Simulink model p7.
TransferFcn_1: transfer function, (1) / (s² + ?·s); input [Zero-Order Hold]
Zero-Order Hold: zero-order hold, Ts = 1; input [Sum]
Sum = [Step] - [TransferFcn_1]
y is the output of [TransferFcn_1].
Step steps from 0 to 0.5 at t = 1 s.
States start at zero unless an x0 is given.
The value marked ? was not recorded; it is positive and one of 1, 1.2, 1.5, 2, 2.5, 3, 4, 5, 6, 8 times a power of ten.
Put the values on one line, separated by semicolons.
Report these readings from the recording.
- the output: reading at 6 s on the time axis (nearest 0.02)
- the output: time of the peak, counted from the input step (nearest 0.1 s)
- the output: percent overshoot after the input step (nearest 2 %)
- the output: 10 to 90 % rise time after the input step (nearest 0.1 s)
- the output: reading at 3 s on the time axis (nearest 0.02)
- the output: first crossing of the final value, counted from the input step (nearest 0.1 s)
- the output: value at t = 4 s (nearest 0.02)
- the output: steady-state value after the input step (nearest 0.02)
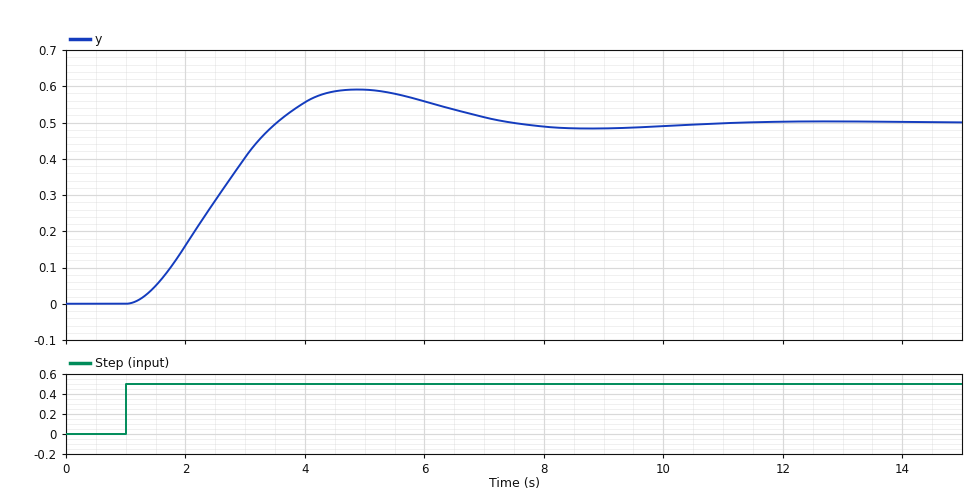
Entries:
0.56; 3.9 s; 18 %; 1.7 s; 0.40; 2.5 s; 0.56; 0.50
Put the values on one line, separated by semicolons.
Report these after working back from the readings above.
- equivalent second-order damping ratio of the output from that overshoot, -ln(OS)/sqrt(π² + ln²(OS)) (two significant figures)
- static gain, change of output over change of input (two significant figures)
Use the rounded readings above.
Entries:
0.48; 1.0
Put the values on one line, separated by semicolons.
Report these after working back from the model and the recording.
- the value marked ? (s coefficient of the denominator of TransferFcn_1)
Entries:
1.5
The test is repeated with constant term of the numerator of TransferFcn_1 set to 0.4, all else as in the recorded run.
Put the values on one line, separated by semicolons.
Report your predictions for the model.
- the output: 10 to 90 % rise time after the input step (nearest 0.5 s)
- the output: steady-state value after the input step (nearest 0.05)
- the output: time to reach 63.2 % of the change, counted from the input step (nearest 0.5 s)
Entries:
5.5 s; 0.50; 3.5 s
